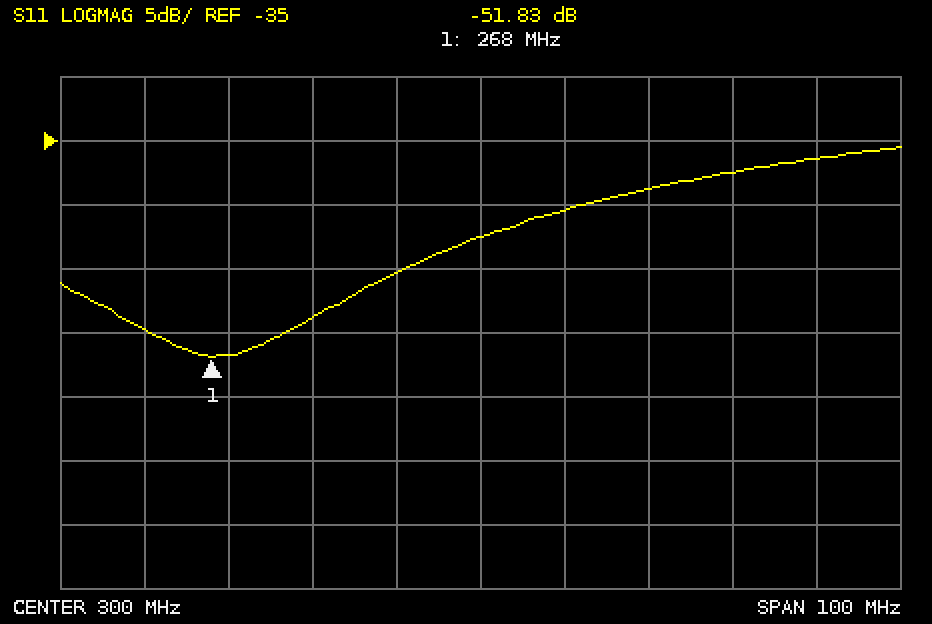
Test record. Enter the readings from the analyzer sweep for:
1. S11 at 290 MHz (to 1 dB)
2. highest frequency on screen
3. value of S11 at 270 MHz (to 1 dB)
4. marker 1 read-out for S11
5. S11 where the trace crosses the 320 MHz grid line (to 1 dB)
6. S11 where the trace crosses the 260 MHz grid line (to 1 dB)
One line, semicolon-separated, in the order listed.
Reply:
-45 dB; 350 MHz; -52 dB; -51.83 dB; -39 dB; -50 dB
